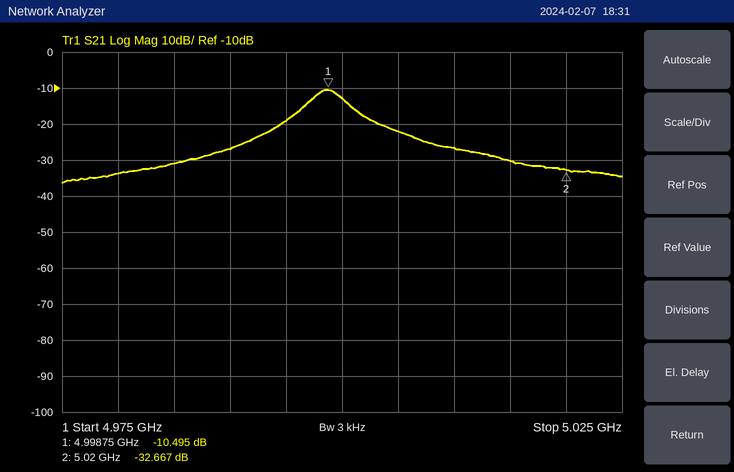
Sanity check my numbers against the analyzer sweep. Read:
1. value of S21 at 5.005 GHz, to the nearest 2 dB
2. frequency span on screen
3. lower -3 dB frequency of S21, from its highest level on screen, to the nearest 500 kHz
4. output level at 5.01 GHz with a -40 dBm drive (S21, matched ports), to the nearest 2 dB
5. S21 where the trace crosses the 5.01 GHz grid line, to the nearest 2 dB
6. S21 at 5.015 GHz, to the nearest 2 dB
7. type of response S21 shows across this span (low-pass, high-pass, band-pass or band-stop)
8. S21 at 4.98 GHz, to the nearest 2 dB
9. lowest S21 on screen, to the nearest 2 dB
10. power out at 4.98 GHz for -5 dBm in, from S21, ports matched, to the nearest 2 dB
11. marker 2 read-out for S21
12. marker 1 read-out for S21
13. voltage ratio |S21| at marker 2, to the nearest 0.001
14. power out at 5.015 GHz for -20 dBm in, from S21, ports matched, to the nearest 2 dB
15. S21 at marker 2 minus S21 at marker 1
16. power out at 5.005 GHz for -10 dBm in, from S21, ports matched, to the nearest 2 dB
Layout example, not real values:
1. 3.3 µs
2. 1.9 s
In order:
1. -22 dB
2. 50 MHz
3. 4.9970 GHz
4. -66 dBm
5. -26 dB
6. -30 dB
7. band-pass
8. -34 dB
9. -36 dB
10. -38 dBm
11. -32.667 dB
12. -10.495 dB
13. 0.023
14. -50 dBm
15. -22.172 dB
16. -32 dBm
